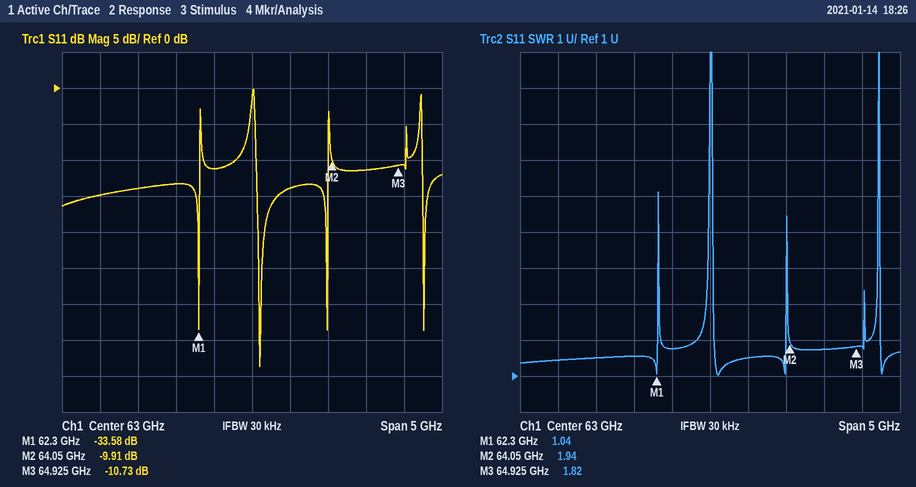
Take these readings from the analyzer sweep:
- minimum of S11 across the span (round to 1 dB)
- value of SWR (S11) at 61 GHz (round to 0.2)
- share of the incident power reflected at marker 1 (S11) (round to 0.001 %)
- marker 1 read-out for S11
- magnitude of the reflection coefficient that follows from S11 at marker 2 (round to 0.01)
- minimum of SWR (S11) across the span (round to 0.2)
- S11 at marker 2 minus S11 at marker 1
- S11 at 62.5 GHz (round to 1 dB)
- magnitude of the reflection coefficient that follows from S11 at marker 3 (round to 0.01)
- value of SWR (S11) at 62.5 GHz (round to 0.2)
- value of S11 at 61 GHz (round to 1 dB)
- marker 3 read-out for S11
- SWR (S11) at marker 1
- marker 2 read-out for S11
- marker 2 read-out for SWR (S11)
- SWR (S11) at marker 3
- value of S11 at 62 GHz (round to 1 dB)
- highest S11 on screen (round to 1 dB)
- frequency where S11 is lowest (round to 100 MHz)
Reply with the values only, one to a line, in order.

-39 dB
1.4
0.044 %
-33.58 dB
0.32
1.0
23.67 dB
-11 dB
0.29
1.8
-15 dB
-10.73 dB
1.04
-9.91 dB
1.94
1.82
-13 dB
0 dB
63.1 GHz
